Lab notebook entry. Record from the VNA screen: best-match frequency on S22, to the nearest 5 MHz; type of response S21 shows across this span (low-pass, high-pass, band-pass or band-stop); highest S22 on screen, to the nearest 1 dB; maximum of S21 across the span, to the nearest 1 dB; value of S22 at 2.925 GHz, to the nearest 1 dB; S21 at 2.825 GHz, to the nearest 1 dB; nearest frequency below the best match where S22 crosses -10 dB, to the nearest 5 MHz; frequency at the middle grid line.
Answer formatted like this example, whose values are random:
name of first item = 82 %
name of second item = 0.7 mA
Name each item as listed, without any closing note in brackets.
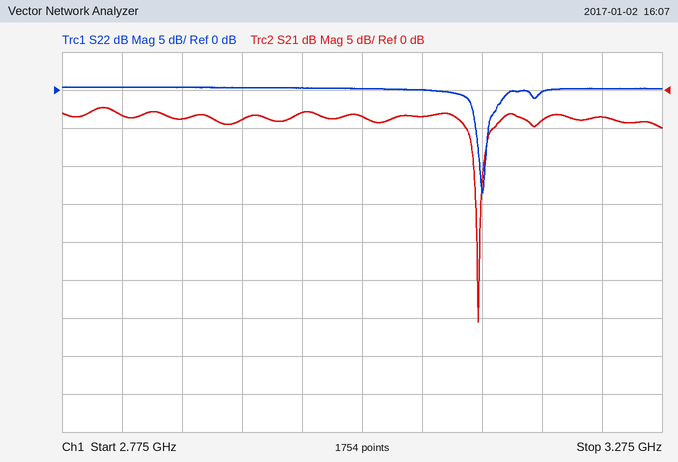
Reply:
best-match frequency on S22, to the nearest 5 MHz = 3.125 GHz
type of response S21 shows across this span = band-stop
highest S22 on screen, to the nearest 1 dB = 0 dB
maximum of S21 across the span, to the nearest 1 dB = -2 dB
value of S22 at 2.925 GHz, to the nearest 1 dB = 0 dB
S21 at 2.825 GHz, to the nearest 1 dB = -3 dB
nearest frequency below the best match where S22 crosses -10 dB, to the nearest 5 MHz = 3.125 GHz
frequency at the middle grid line = 3.025 GHz
